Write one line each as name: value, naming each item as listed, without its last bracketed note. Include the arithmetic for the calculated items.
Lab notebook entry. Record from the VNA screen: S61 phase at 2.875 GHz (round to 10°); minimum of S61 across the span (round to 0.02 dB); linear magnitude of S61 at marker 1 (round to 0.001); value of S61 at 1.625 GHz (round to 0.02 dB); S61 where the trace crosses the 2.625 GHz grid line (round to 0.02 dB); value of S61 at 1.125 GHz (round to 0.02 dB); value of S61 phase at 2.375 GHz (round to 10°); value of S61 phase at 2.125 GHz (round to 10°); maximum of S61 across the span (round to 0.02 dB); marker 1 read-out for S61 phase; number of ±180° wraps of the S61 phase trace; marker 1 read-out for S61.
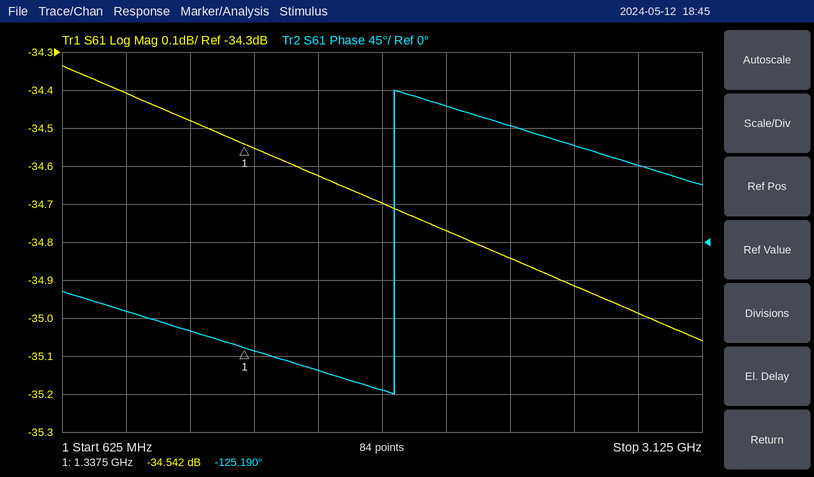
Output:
S61 phase at 2.875 GHz: 90°
minimum of S61 across the span: -35.06 dB
linear magnitude of S61 at marker 1: 10^(-34.542/20) ≈ 0.019
value of S61 at 1.625 GHz: -34.62 dB
S61 where the trace crosses the 2.625 GHz grid line: -34.92 dB
value of S61 at 1.125 GHz: -34.48 dB
value of S61 phase at 2.375 GHz: 140°
value of S61 phase at 2.125 GHz: 160°
maximum of S61 across the span: -34.34 dB
marker 1 read-out for S61 phase: -125.190°
number of ±180° wraps of the S61 phase trace: 1
marker 1 read-out for S61: -34.542 dB
